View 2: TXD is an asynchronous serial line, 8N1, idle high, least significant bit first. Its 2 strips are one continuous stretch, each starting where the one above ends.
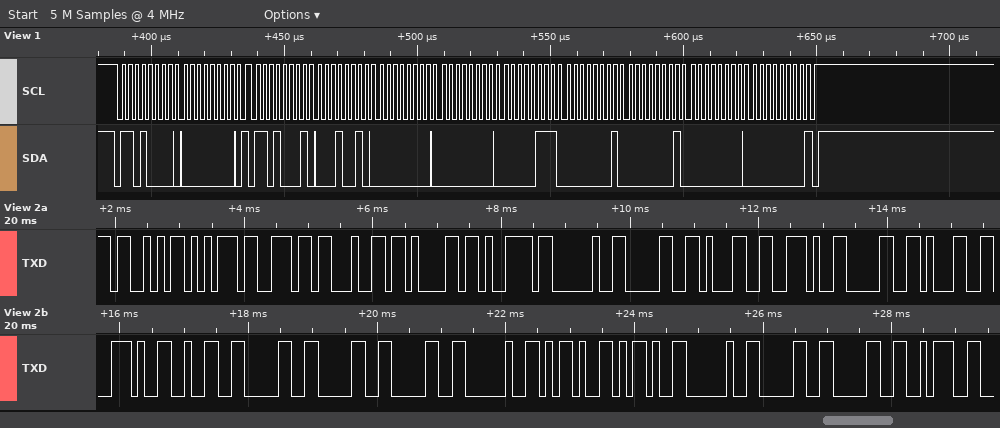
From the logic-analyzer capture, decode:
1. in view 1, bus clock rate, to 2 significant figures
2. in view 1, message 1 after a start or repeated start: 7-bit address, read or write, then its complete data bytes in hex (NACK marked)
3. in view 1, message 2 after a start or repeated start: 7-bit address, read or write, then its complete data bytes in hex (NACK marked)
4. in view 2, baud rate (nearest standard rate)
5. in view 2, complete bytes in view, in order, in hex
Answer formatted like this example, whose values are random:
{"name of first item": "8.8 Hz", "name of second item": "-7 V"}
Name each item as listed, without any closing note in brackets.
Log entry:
{"in view 1, bus clock rate, to 2 significant figures": "400 kHz", "in view 1, message 1 after a start or repeated start: 7-bit address, read or write, then its complete data bytes in hex": "0x68 write: 00", "in view 1, message 2 after a start or repeated start: 7-bit address, read or write, then its complete data bytes in hex": "0x68 read: 12 00 00 07 01 01 00 00 NACK", "in view 2, baud rate": "9600 baud", "in view 2, complete bytes in view, in order, in hex": "53 75 6E 64 61 79 20 30 31 2E 30 31 2E 32 30 30 30 20 2D 2D 20 30 30 3A"}
